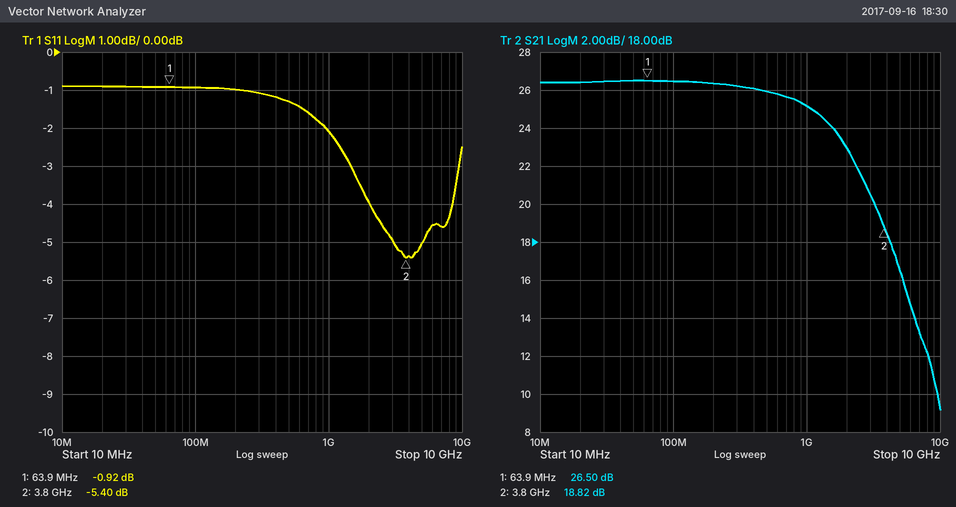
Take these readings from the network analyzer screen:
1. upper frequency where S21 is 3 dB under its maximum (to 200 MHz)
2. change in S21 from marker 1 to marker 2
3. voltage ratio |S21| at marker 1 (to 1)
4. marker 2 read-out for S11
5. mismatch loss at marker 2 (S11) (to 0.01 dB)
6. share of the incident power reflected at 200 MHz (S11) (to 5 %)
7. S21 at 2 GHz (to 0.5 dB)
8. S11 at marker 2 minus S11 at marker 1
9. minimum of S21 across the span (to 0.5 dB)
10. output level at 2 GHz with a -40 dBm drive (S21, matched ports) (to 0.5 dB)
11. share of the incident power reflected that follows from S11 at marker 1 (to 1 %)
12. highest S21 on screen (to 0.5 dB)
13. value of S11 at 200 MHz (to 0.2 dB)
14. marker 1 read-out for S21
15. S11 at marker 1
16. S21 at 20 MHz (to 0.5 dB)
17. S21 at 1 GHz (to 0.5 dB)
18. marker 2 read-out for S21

1.8 GHz
-7.68 dB
21
-5.40 dB
1.48 dB
80 %
23.0 dB
-4.48 dB
9.0 dB
-17.0 dBm
81 %
26.5 dB
-1.0 dB
26.50 dB
-0.92 dB
26.5 dB
25.0 dB
18.82 dB
